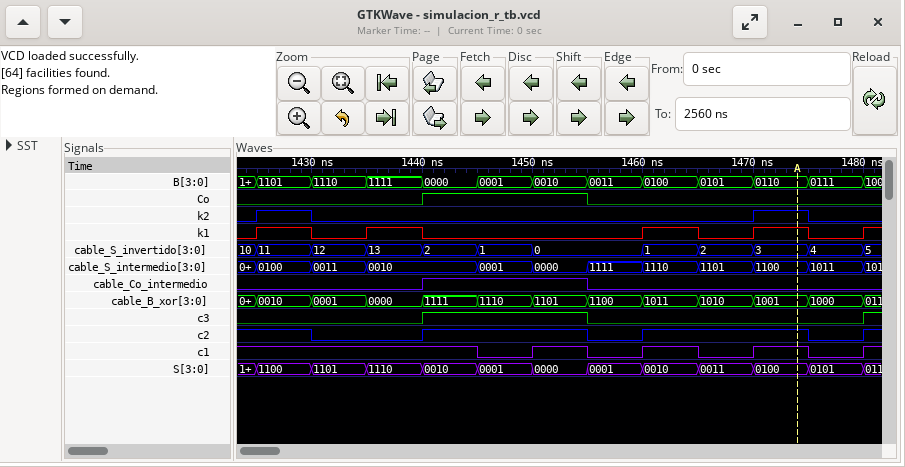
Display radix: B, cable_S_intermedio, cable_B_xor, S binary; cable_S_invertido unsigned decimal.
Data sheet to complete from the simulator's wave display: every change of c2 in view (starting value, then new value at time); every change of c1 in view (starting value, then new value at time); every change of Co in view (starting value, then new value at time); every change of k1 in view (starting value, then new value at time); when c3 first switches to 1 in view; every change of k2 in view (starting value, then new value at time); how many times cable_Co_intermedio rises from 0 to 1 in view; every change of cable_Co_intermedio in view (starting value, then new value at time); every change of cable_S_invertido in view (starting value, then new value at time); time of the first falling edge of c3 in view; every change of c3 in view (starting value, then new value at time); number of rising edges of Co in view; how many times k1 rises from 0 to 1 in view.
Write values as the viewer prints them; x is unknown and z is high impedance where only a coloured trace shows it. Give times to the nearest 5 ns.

1, 0 at 1430 ns, 1 at 1440 ns, 0 at 1455 ns, 1 at 1460 ns, 0 at 1475 ns, 1 at 1480 ns
1, 0 at 1445 ns, 1 at 1450 ns, 0 at 1455 ns, 1 at 1460 ns, 0 at 1465 ns, 1 at 1470 ns, 0 at 1475 ns, 1 at 1480 ns
0, 1 at 1440 ns, 0 at 1455 ns
0, 1 at 1425 ns, 0 at 1430 ns, 1 at 1435 ns, 0 at 1440 ns, 1 at 1460 ns, 0 at 1465 ns, 1 at 1470 ns, 0 at 1475 ns, 1 at 1480 ns
1440 ns
0, 1 at 1425 ns, 0 at 1430 ns, 1 at 1470 ns, 0 at 1475 ns
1
0, 1 at 1440 ns, 0 at 1455 ns
10, 11 at 1425 ns, 12 at 1430 ns, 13 at 1435 ns, 2 at 1440 ns, 1 at 1445 ns, 0 at 1450 ns, 1 at 1460 ns, 2 at 1465 ns, 3 at 1470 ns, 4 at 1475 ns, 5 at 1480 ns
1455 ns
0, 1 at 1440 ns, 0 at 1455 ns, 1 at 1480 ns
1
5
